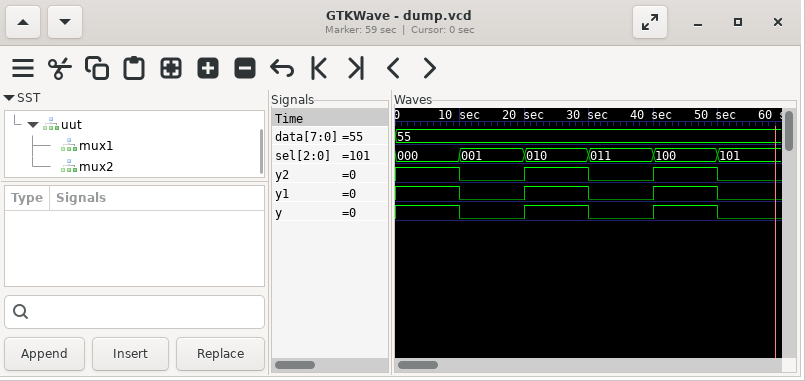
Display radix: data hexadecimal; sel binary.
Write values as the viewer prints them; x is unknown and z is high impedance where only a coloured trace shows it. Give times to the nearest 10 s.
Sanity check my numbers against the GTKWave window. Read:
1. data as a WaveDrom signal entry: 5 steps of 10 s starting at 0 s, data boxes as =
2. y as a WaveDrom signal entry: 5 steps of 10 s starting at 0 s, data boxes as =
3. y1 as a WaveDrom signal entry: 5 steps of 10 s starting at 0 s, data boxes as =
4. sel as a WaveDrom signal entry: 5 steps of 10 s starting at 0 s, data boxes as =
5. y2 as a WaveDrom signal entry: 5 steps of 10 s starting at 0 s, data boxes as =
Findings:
{name: 'data', wave: '=....', data: '55'}
{name: 'y', wave: '10101'}
{name: 'y1', wave: '10101'}
{name: 'sel', wave: '=====', data: '000 001 010 011 100'}
{name: 'y2', wave: '10101'}
